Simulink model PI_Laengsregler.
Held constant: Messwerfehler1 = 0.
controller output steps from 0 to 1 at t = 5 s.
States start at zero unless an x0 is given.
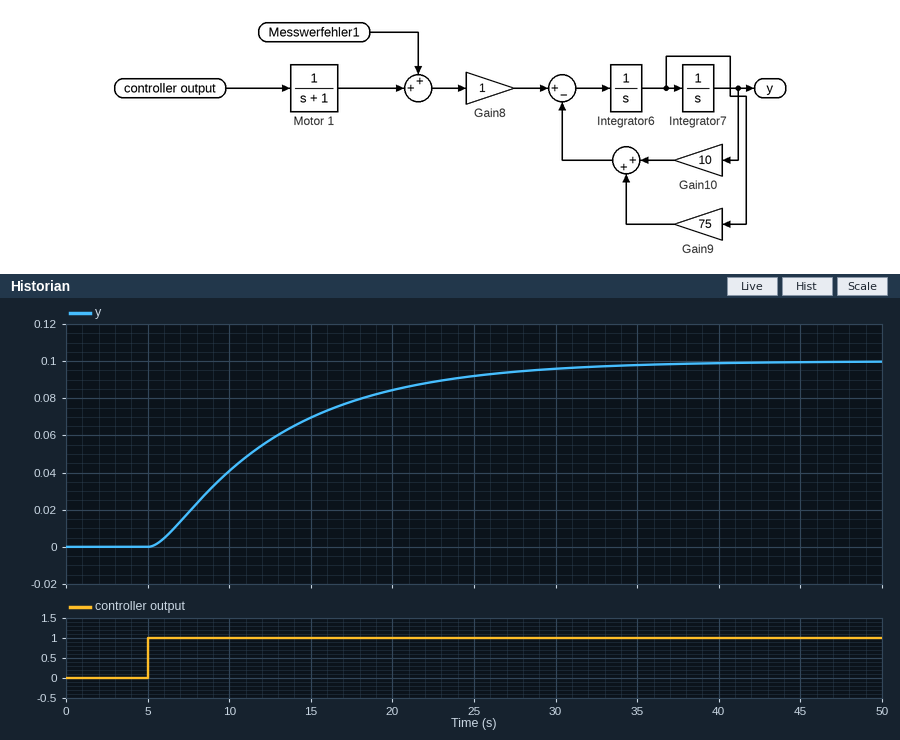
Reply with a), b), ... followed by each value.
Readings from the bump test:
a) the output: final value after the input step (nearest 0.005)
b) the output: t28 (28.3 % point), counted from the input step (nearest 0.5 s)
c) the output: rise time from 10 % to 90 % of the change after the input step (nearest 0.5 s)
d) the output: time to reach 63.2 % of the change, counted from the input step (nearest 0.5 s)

a) 0.100
b) 3.5 s
c) 16.5 s
d) 8.5 s
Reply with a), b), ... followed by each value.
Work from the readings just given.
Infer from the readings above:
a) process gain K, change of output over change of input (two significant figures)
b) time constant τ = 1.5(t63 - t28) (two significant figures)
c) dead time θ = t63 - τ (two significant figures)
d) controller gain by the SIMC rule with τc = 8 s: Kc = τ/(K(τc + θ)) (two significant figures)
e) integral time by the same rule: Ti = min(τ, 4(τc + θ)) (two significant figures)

a) 0.10
b) 7.5 s
c) 1.0 s
d) 8.3
e) 7.5 s
